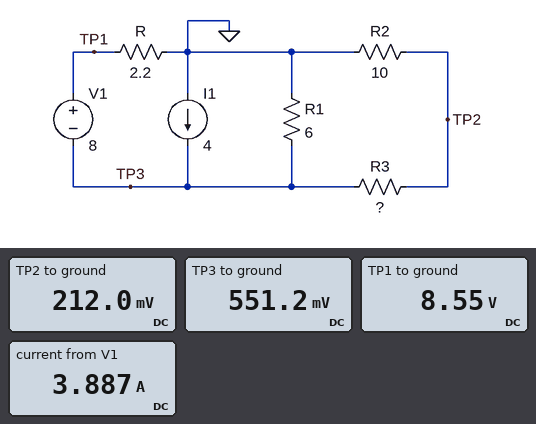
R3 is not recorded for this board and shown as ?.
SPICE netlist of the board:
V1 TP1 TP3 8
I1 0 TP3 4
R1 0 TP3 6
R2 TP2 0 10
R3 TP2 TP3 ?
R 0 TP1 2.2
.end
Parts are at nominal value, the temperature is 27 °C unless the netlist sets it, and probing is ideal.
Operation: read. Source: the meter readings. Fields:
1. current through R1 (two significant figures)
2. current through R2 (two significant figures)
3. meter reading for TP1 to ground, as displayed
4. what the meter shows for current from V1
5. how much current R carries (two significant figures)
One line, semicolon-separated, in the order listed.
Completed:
92 mA; 21 mA; 8.55 V; 3.887 A; 3.9 A
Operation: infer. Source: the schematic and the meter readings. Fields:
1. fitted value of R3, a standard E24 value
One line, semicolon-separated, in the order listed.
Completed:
16 Ω
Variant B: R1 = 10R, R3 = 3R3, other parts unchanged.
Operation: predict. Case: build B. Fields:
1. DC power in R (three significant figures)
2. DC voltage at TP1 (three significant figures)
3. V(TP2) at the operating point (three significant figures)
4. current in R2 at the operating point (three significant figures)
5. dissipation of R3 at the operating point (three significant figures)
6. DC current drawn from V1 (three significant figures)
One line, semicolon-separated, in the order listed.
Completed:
33.4 W; 8.58 V; 434 mV; 43.4 mA; 6.22 mW; 3.90 A
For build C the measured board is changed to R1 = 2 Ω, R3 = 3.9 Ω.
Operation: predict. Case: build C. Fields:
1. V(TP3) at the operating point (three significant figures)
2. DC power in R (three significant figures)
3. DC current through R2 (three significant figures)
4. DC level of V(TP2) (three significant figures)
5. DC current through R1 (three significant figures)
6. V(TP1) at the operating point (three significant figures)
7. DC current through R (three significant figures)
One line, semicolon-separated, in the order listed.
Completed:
354 mV; 31.7 W; 25.5 mA; 255 mV; 177 mA; 8.35 V; 3.80 A
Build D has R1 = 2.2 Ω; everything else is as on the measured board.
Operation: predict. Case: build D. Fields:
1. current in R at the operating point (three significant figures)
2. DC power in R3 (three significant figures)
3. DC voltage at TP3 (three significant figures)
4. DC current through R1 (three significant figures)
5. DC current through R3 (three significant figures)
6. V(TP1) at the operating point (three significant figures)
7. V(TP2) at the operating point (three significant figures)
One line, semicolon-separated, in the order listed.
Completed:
3.81 A; 3.49 mW; 384 mV; 174 mA; 14.8 mA; 8.38 V; 148 mV
